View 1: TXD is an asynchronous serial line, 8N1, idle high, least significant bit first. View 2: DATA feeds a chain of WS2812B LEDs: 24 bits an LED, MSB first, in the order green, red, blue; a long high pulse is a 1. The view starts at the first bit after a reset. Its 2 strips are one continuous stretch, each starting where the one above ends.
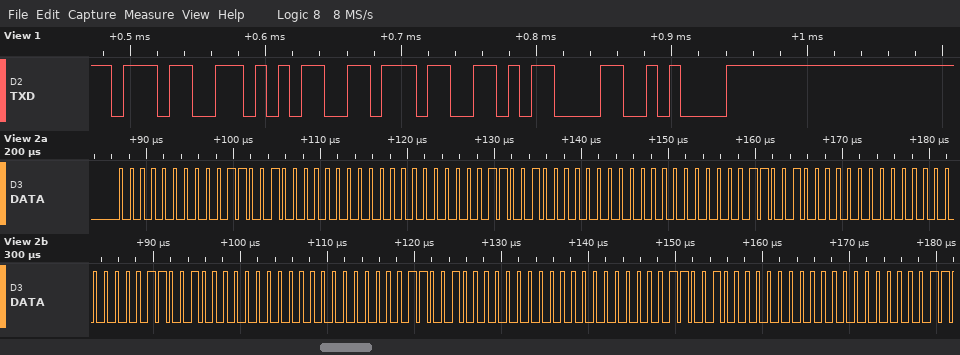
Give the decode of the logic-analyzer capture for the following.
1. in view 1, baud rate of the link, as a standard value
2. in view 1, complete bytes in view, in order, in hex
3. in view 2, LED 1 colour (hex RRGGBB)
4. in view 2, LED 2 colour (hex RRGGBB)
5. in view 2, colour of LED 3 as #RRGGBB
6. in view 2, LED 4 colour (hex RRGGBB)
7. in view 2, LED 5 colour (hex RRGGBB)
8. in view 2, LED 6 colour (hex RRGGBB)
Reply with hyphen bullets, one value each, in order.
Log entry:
- 115200 baud
- 37 35 37 0D 0A
- #320000
- #320000
- #320000
- #320000
- #320000
- #320000
